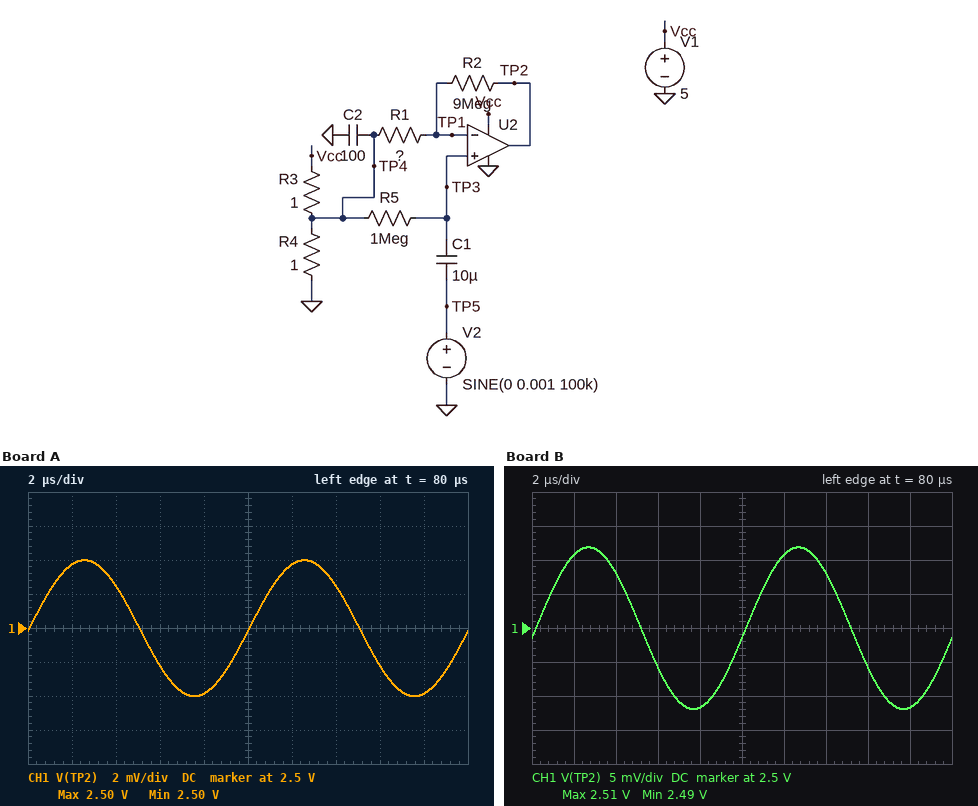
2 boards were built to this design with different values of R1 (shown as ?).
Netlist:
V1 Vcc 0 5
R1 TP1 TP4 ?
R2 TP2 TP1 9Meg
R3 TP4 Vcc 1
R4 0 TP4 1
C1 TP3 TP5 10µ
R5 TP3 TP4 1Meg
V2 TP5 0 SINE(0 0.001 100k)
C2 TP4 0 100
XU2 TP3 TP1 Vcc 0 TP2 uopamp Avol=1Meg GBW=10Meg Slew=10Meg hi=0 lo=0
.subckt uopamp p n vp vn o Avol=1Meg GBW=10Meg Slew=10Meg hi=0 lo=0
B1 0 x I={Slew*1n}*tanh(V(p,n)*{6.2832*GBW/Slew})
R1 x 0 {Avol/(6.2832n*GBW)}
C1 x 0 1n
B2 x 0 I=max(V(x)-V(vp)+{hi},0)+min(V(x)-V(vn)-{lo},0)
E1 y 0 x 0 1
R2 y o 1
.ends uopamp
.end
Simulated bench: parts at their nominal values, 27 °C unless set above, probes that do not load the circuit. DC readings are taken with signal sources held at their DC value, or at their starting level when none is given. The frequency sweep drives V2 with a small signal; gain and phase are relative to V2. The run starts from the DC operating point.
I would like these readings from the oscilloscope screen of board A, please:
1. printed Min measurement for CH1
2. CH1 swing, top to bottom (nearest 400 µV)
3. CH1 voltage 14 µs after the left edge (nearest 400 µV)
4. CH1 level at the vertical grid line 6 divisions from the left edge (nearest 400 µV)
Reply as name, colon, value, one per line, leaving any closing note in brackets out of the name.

printed Min measurement for CH1: 2.50 V
CH1 swing, top to bottom: 8.0 mV
CH1 voltage 14 µs after the left edge: 2.5024 V
CH1 level at the vertical grid line 6 divisions from the left edge: 2.5036 V
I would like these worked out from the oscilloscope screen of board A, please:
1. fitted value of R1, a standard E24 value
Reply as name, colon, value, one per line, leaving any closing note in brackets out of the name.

fitted value of R1, a standard E24 value: 3 MΩ
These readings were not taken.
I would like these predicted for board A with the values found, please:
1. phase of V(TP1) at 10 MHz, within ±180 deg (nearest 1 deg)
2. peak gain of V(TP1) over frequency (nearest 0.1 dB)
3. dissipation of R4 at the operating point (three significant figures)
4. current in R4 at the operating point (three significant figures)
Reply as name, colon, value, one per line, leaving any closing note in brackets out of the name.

phase of V(TP1) at 10 MHz, within ±180 deg: -76 deg
peak gain of V(TP1) over frequency: 0 dB
dissipation of R4 at the operating point: 6.25 W
current in R4 at the operating point: 2.50 A
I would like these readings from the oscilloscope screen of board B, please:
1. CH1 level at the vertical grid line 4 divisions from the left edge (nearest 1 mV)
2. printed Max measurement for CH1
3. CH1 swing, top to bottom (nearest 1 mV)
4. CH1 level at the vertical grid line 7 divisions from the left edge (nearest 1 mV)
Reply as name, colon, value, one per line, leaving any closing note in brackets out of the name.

CH1 level at the vertical grid line 4 divisions from the left edge: 2.488 V
printed Max measurement for CH1: 2.51 V
CH1 swing, top to bottom: 24 mV
CH1 level at the vertical grid line 7 divisions from the left edge: 2.508 V
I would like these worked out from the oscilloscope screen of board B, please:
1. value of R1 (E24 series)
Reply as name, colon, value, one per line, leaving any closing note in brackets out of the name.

value of R1: 820 kΩ
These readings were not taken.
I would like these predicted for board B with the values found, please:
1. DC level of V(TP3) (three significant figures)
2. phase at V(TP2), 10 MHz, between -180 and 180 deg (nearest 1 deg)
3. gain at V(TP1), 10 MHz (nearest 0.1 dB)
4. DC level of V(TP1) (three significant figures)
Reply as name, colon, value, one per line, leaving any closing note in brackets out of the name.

DC level of V(TP3): 2.50 V
phase at V(TP2), 10 MHz, between -180 and 180 deg: -85 deg
gain at V(TP1), 10 MHz: -21.6 dB
DC level of V(TP1): 2.50 V
